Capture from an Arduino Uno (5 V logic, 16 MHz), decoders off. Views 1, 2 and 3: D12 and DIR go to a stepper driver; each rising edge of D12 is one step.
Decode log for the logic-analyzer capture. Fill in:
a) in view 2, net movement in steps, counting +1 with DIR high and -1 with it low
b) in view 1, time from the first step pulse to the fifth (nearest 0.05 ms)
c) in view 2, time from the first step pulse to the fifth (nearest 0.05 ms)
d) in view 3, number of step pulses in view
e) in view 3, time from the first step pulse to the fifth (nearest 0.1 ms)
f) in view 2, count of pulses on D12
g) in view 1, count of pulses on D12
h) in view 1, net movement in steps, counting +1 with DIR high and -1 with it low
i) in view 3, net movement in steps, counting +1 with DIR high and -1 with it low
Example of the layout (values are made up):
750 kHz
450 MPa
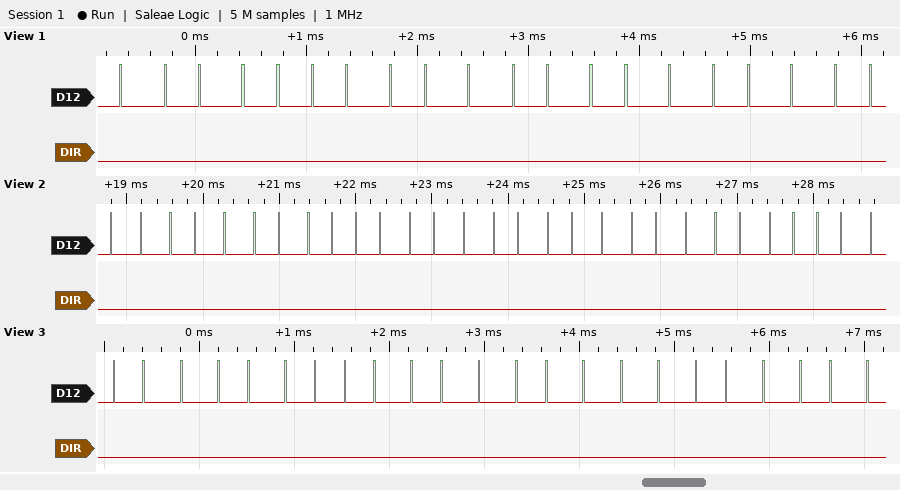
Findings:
-29
1.40 ms
1.50 ms
23
1.4 ms
29
20
-20
-23
